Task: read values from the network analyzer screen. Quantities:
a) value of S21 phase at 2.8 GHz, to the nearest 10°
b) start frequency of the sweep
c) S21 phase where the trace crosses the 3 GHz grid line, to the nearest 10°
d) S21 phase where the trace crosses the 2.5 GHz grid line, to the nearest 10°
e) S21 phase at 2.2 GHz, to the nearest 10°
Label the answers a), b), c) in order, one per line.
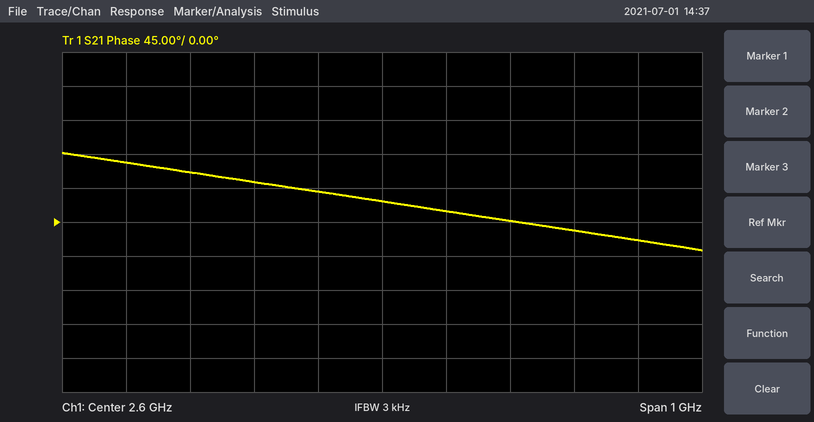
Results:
a) 0°
b) 2.1 GHz
c) -20°
d) 40°
e) 80°
